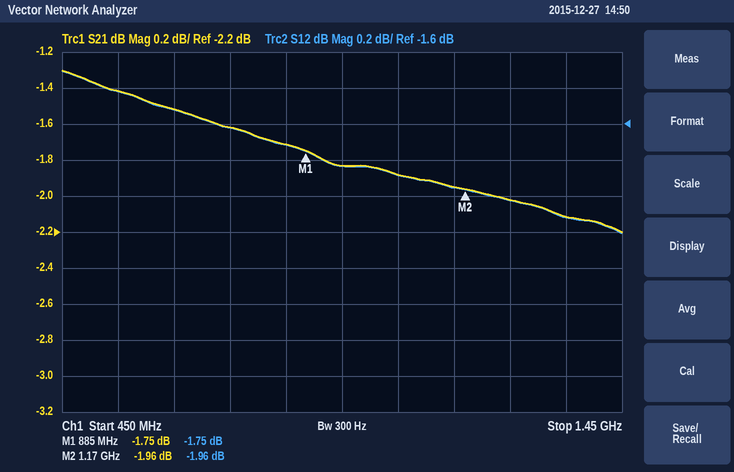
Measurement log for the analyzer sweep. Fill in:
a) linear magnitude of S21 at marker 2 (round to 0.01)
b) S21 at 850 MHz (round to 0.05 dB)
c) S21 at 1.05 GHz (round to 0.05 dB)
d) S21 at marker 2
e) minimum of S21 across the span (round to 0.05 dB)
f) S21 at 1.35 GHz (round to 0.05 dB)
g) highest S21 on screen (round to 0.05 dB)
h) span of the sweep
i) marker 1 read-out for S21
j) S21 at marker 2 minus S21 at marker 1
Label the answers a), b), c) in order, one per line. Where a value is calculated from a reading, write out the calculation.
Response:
a) 10^(-1.96/20) ≈ 0.80
b) -1.70 dB
c) -1.90 dB
d) -1.96 dB
e) -2.20 dB
f) -2.10 dB
g) -1.30 dB
h) 1 GHz
i) -1.75 dB
j) -1.96 − (-1.75) = -0.21 dB
